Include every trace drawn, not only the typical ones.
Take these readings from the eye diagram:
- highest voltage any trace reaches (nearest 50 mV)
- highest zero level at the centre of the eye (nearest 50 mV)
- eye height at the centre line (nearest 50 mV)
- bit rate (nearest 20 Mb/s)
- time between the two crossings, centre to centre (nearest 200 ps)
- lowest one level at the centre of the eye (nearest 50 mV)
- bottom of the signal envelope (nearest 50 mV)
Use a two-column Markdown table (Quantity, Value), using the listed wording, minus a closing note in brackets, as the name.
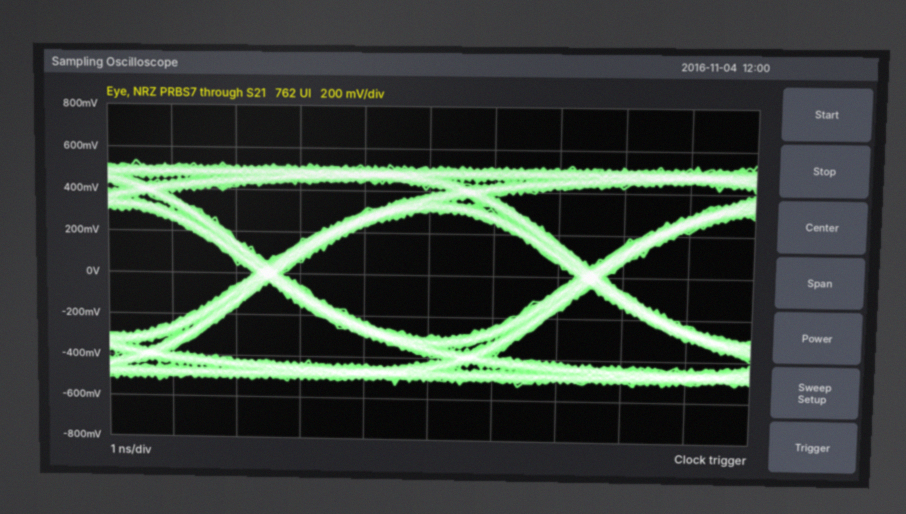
| Quantity | Value |
|---|---|
| highest voltage any trace reaches | 550 mV |
| highest zero level at the centre of the eye | -300 mV |
| eye height at the centre line | 600 mV |
| bit rate | 200 Mb/s |
| time between the two crossings, centre to centre | 5.0 ns |
| lowest one level at the centre of the eye | 300 mV |
| bottom of the signal envelope | -550 mV |
